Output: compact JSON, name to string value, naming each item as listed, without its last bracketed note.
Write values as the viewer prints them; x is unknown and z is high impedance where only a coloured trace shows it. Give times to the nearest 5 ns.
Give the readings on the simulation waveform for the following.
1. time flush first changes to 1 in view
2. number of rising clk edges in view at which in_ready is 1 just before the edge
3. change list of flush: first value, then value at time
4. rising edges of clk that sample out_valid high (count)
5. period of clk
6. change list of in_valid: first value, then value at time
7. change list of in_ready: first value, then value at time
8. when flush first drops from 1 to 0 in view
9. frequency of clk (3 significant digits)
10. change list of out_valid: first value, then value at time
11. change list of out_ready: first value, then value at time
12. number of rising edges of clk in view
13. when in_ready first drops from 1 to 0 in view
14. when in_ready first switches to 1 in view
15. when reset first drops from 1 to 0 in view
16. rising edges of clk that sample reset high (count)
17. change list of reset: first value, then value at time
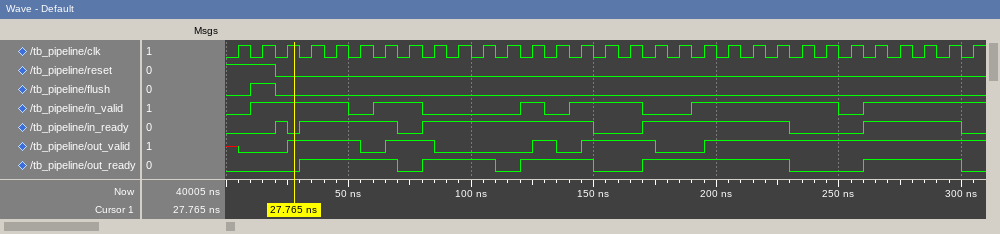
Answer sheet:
{"time flush first changes to 1 in view": "10 ns", "number of rising clk edges in view at which in_ready is 1 just before the edge": "22", "change list of flush: first value, then value at time": "0, 1 at 10 ns, 0 at 20 ns", "rising edges of clk that sample out_valid high": "20", "period of clk": "10 ns", "change list of in_valid: first value, then value at time": "0, 1 at 10 ns, 0 at 50 ns, 1 at 60 ns, 0 at 80 ns, 1 at 120 ns, 0 at 130 ns, 1 at 140 ns, 0 at 170 ns, 1 at 190 ns, 0 at 250 ns, 1 at 260 ns", "change list of in_ready: first value, then value at time": "0, 1 at 20 ns, 0 at 25 ns, 1 at 30 ns, 0 at 70 ns, 1 at 80 ns, 0 at 150 ns, 1 at 170 ns, 0 at 230 ns, 1 at 260 ns, 0 at 300 ns", "when flush first drops from 1 to 0 in view": "20 ns", "frequency of clk": "100 MHz", "change list of out_valid: first value, then value at time": "x, 0 at 5 ns, 1 at 25 ns, 0 at 55 ns, 1 at 65 ns, 0 at 85 ns, 1 at 125 ns, 0 at 135 ns, 1 at 145 ns, 0 at 175 ns, 1 at 195 ns", "change list of out_ready: first value, then value at time": "0, 1 at 30 ns, 0 at 70 ns, 1 at 80 ns, 0 at 110 ns, 1 at 120 ns, 0 at 150 ns, 1 at 170 ns, 0 at 230 ns, 1 at 260 ns, 0 at 300 ns", "number of rising edges of clk in view": "31", "when in_ready first drops from 1 to 0 in view": "25 ns", "when in_ready first switches to 1 in view": "20 ns", "when reset first drops from 1 to 0 in view": "20 ns", "rising edges of clk that sample reset high": "2", "change list of reset: first value, then value at time": "1, 0 at 20 ns"}
